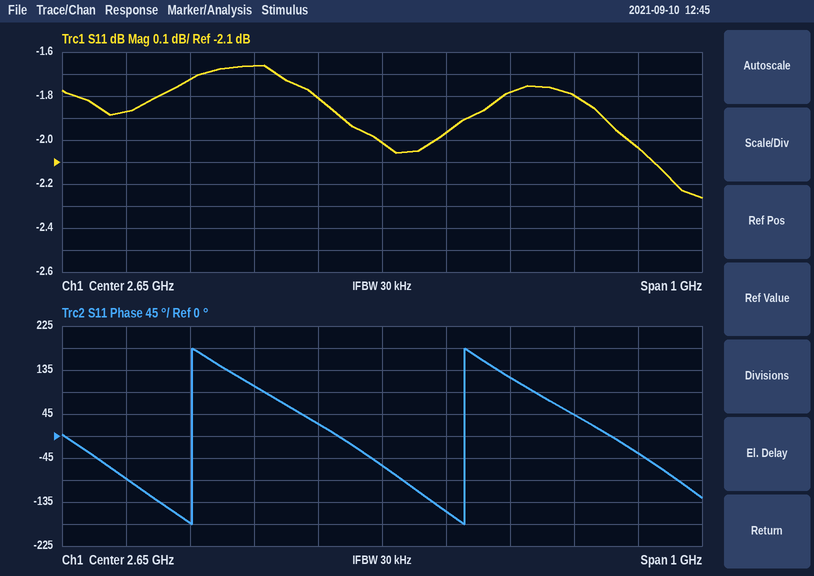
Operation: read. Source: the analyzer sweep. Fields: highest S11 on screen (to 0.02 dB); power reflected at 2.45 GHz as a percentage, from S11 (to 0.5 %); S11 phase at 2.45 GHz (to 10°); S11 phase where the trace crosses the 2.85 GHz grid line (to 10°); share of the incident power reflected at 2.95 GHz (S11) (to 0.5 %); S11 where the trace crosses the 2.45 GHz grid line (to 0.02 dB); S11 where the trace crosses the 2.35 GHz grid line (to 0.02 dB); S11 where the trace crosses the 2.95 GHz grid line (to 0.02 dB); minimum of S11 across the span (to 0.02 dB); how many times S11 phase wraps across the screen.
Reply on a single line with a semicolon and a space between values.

-1.66 dB; 68.0 %; 100°; 120°; 66.0 %; -1.66 dB; -1.72 dB; -1.80 dB; -2.26 dB; 2
